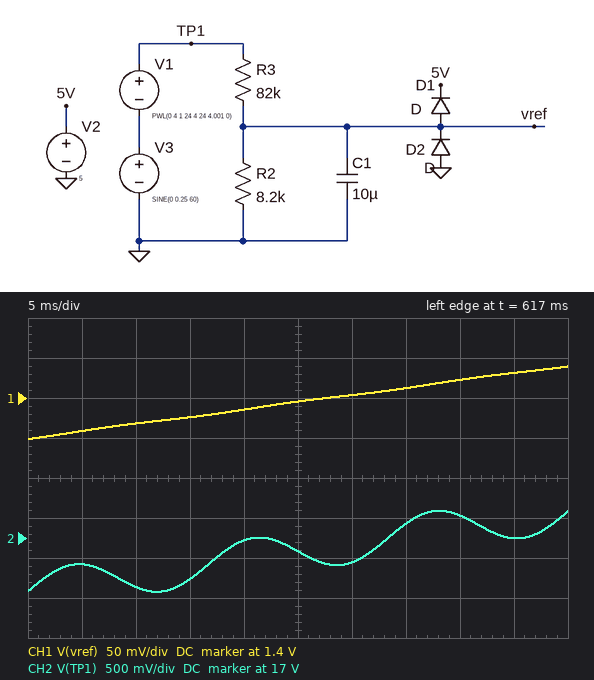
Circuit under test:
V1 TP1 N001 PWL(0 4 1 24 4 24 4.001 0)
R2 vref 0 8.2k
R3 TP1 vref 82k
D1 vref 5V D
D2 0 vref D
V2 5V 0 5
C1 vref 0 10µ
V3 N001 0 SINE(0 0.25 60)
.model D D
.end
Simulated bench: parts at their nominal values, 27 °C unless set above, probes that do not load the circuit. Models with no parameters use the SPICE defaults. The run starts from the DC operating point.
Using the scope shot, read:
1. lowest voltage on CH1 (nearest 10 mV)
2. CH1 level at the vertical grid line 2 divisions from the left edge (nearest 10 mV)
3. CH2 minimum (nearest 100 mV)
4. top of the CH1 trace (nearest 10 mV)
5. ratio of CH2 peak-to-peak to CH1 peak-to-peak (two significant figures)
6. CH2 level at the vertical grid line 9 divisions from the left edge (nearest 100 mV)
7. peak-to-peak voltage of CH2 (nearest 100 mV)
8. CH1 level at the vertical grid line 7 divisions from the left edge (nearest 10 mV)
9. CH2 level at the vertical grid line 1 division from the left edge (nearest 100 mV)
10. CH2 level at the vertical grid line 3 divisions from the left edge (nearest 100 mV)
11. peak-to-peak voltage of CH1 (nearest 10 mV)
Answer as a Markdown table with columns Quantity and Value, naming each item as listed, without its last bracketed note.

| Quantity | Value |
|---|---|
| lowest voltage on CH1 | 1.35 V |
| CH1 level at the vertical grid line 2 divisions from the left edge | 1.37 V |
| CH2 minimum | 16.3 V |
| top of the CH1 trace | 1.44 V |
| ratio of CH2 peak-to-peak to CH1 peak-to-peak | 11 |
| CH2 level at the vertical grid line 9 divisions from the left edge | 17.0 V |
| peak-to-peak voltage of CH2 | 1.0 V |
| CH1 level at the vertical grid line 7 divisions from the left edge | 1.41 V |
| CH2 level at the vertical grid line 1 division from the left edge | 16.7 V |
| CH2 level at the vertical grid line 3 divisions from the left edge | 16.5 V |
| peak-to-peak voltage of CH1 | 90 mV |
